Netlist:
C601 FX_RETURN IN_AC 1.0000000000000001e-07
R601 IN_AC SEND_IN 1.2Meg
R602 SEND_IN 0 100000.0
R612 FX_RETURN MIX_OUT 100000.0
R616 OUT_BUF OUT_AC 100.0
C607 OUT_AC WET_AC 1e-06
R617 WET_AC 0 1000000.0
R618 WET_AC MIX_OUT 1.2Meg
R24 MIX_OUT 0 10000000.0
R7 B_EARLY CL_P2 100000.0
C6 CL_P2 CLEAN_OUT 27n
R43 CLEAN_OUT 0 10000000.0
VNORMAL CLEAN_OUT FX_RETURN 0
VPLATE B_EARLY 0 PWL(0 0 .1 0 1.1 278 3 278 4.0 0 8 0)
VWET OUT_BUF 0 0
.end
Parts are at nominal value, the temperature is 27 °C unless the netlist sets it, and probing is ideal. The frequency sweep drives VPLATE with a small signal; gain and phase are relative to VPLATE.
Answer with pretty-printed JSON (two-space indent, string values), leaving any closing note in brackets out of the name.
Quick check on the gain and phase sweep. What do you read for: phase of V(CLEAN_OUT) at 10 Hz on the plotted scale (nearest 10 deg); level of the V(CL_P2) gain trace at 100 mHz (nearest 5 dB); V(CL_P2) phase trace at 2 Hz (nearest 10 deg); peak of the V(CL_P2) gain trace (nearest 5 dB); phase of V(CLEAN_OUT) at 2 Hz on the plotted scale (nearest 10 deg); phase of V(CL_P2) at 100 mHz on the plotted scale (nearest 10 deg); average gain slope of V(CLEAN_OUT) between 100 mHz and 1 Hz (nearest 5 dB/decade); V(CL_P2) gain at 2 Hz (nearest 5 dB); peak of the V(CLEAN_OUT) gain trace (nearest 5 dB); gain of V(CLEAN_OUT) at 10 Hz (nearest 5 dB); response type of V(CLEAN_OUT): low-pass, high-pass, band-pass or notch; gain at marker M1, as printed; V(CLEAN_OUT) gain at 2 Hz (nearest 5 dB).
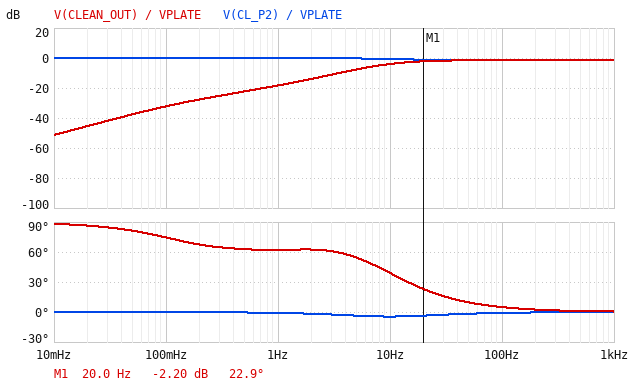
{
  "phase of V(CLEAN_OUT) at 10 Hz on the plotted scale": "40 deg",
  "level of the V(CL_P2) gain trace at 100 mHz": "0 dB",
  "V(CL_P2) phase trace at 2 Hz": "0 deg",
  "peak of the V(CL_P2) gain trace": "0 dB",
  "phase of V(CLEAN_OUT) at 2 Hz on the plotted scale": "60 deg",
  "phase of V(CL_P2) at 100 mHz on the plotted scale": "0 deg",
  "average gain slope of V(CLEAN_OUT) between 100 mHz and 1 Hz": "15 dB/decade",
  "V(CL_P2) gain at 2 Hz": "0 dB",
  "peak of the V(CLEAN_OUT) gain trace": "0 dB",
  "gain of V(CLEAN_OUT) at 10 Hz": "-5 dB",
  "response type of V(CLEAN_OUT): low-pass, high-pass, band-pass or notch": "high-pass",
  "gain at marker M1, as printed": "-2.20 dB",
  "V(CLEAN_OUT) gain at 2 Hz": "-15 dB"
}
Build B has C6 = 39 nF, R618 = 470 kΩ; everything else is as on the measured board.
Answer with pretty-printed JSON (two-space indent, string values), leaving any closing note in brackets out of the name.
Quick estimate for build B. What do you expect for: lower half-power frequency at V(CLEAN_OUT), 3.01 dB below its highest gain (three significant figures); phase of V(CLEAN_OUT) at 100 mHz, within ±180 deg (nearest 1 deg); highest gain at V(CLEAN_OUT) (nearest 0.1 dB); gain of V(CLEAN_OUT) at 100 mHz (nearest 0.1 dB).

{
  "lower half-power frequency at V(CLEAN_OUT), 3.01 dB below its highest gain": "9.01 Hz",
  "phase of V(CLEAN_OUT) at 100 mHz, within ±180 deg": "70 deg",
  "highest gain at V(CLEAN_OUT)": "-2.1 dB",
  "gain of V(CLEAN_OUT) at 100 mHz": "-31.7 dB"
}
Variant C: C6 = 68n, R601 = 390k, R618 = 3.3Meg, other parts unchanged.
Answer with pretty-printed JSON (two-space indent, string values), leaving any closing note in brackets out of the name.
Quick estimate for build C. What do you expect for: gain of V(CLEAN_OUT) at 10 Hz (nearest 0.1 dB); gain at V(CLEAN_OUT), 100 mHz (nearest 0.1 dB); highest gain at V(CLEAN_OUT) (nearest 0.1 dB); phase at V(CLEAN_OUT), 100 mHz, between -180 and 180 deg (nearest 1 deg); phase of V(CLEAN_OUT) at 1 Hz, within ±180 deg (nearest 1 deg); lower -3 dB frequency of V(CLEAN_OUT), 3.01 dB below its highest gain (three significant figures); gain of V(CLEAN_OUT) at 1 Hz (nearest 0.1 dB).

{
  "gain of V(CLEAN_OUT) at 10 Hz": "-3.3 dB",
  "gain at V(CLEAN_OUT), 100 mHz": "-20.6 dB",
  "highest gain at V(CLEAN_OUT)": "-2.0 dB",
  "phase at V(CLEAN_OUT), 100 mHz, between -180 and 180 deg": "73 deg",
  "phase of V(CLEAN_OUT) at 1 Hz, within ±180 deg": "31 deg",
  "lower -3 dB frequency of V(CLEAN_OUT), 3.01 dB below its highest gain": "5.36 Hz",
  "gain of V(CLEAN_OUT) at 1 Hz": "-9.1 dB"
}
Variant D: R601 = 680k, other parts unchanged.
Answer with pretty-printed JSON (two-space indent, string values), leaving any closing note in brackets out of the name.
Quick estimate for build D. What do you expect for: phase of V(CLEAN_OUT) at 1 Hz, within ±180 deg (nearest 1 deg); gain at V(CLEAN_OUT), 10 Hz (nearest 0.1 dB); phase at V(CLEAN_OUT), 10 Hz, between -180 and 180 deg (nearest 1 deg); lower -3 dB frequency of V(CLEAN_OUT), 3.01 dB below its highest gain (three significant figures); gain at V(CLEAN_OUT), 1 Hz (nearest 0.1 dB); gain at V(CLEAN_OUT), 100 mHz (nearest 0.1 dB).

{
  "phase of V(CLEAN_OUT) at 1 Hz, within ±180 deg": "56 deg",
  "gain at V(CLEAN_OUT), 10 Hz": "-5.4 dB",
  "phase at V(CLEAN_OUT), 10 Hz, between -180 and 180 deg": "43 deg",
  "lower -3 dB frequency of V(CLEAN_OUT), 3.01 dB below its highest gain": "11.5 Hz",
  "gain at V(CLEAN_OUT), 1 Hz": "-18.4 dB",
  "gain at V(CLEAN_OUT), 100 mHz": "-32.2 dB"
}
